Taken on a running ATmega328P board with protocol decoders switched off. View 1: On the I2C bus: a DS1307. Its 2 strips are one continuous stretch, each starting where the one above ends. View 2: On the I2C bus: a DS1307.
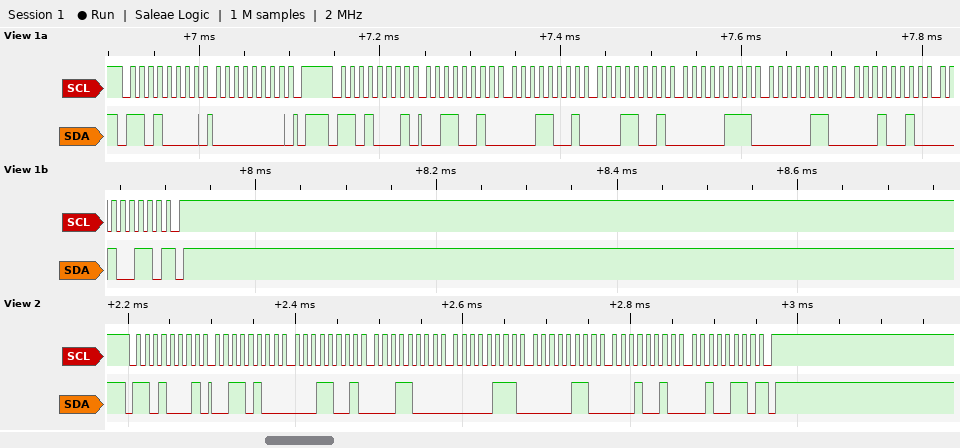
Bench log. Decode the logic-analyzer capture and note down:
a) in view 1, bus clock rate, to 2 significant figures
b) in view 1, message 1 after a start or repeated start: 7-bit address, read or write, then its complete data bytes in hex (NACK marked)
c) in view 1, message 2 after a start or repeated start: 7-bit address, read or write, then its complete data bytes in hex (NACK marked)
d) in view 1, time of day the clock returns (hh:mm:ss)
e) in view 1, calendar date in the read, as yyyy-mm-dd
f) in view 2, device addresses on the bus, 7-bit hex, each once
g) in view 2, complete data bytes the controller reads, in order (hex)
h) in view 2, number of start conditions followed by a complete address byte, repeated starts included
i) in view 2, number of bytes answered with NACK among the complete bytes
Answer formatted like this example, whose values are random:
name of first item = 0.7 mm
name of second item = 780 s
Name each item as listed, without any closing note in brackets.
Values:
in view 1, bus clock rate, to 2 significant figures = 100 kHz
in view 1, message 1 after a start or repeated start: 7-bit address, read or write, then its complete data bytes in hex = 0x68 write: 00
in view 1, message 2 after a start or repeated start: 7-bit address, read or write, then its complete data bytes in hex = 0x68 read: 32 19 19 07 06 12 26 NACK
in view 1, time of day the clock returns = 19:19:32
in view 1, calendar date in the read, as yyyy-mm-dd = 2026-12-06
in view 2, device addresses on the bus, 7-bit hex, each once = 0x68
in view 2, complete data bytes the controller reads, in order = 34 19 18 07 06 12 26
in view 2, number of start conditions followed by a complete address byte, repeated starts included = 1
in view 2, number of bytes answered with NACK among the complete bytes = 1
